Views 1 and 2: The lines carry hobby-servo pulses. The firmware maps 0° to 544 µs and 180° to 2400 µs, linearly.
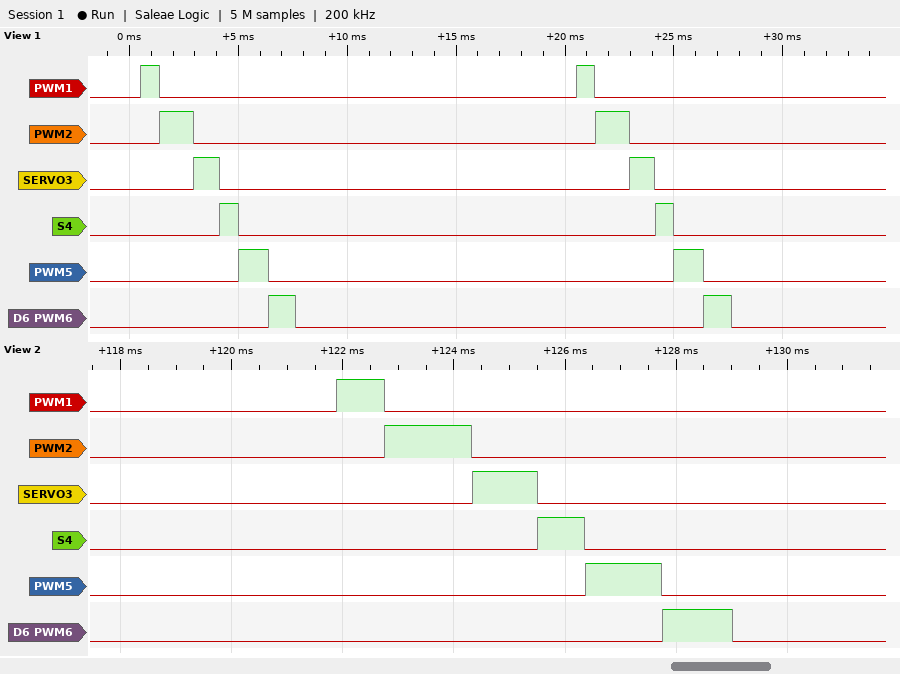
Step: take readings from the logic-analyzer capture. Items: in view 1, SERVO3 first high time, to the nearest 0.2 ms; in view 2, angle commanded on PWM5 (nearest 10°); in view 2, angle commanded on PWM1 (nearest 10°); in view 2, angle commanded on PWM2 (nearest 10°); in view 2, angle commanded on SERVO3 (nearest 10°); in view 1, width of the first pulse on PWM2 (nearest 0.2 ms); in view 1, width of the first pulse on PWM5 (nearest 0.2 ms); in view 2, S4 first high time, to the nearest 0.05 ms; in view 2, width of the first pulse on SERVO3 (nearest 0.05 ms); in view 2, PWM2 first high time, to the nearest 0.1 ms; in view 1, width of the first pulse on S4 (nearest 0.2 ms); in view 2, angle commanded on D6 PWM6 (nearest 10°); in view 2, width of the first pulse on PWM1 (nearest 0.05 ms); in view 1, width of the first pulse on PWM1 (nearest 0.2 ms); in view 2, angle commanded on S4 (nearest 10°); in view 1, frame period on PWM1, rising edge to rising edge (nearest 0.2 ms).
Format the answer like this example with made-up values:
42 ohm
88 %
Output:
1.2 ms
80°
30°
100°
60°
1.6 ms
1.4 ms
0.85 ms
1.15 ms
1.6 ms
0.8 ms
70°
0.85 ms
0.8 ms
30°
20.0 ms
